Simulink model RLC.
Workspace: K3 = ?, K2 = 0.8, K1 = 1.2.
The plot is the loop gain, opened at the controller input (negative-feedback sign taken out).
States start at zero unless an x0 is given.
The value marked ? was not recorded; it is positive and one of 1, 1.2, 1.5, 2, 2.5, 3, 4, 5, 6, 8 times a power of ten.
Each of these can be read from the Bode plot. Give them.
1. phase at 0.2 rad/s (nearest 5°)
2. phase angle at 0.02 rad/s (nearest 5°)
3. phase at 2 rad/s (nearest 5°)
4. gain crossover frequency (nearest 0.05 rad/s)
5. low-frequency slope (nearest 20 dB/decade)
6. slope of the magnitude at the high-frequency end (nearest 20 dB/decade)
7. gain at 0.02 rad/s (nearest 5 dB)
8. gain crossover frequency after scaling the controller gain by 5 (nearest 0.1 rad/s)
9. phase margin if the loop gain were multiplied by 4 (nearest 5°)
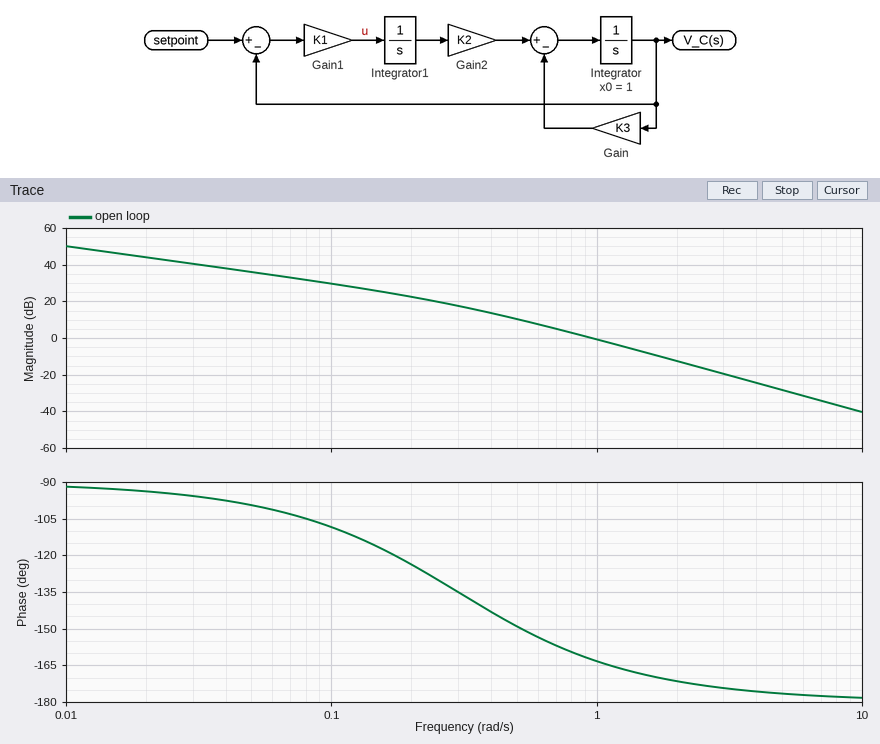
-125°
-95°
-170°
0.95 rad/s
-20 dB/decade
-40 dB/decade
45 dB
2.2 rad/s
10°
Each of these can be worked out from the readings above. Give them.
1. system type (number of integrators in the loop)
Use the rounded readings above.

1
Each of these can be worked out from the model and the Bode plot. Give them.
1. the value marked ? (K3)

0.3
